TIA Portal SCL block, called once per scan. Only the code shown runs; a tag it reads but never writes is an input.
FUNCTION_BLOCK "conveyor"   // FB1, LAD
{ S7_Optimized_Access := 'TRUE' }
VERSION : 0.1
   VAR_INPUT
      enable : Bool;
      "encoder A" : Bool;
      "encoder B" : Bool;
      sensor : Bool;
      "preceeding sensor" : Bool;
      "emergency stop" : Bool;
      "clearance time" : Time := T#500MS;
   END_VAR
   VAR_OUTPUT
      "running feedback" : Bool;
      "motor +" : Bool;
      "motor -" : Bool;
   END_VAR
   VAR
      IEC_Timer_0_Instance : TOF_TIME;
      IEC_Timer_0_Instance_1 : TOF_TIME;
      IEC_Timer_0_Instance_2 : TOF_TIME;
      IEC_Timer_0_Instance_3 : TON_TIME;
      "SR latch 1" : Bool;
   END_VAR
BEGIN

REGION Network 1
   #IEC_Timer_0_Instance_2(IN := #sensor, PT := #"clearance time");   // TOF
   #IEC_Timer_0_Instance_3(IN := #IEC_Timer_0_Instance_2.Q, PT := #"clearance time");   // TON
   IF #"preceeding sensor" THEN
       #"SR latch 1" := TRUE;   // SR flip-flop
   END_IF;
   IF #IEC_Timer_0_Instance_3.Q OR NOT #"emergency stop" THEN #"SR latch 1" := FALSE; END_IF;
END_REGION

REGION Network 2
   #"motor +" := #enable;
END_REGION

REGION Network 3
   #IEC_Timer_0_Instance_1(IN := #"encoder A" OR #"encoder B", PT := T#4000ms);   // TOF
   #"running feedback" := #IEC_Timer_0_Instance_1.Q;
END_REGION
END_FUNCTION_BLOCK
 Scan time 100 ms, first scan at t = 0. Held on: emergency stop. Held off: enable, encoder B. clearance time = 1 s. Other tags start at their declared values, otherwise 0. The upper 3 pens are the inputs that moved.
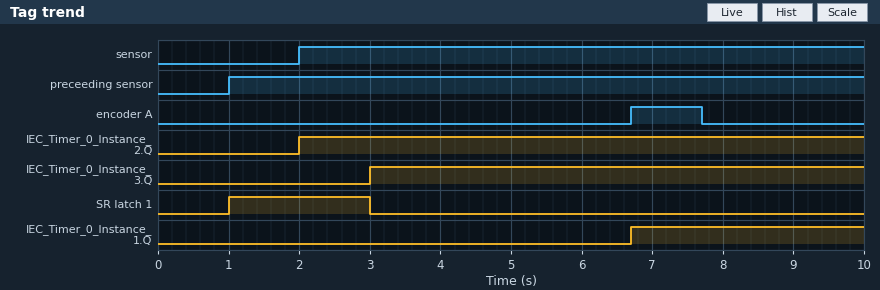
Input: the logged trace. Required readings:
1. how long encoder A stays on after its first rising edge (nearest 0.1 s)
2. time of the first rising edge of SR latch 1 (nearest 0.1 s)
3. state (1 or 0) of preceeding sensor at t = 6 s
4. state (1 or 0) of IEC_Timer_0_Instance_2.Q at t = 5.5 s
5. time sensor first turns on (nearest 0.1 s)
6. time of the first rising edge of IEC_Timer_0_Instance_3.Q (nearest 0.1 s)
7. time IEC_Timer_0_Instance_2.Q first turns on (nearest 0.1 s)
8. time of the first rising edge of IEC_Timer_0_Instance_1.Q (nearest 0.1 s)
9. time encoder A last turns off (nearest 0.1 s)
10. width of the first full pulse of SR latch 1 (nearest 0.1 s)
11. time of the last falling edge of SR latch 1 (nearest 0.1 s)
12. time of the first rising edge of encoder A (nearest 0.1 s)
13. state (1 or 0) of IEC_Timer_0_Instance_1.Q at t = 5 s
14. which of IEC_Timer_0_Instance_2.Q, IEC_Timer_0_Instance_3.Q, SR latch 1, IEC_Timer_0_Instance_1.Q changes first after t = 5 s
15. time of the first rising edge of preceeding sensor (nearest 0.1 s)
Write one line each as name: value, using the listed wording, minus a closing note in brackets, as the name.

how long encoder A stays on after its first rising edge: 1.0 s
time of the first rising edge of SR latch 1: 1.0 s
state (1 or 0) of preceeding sensor at t = 6 s: 1
state (1 or 0) of IEC_Timer_0_Instance_2.Q at t = 5.5 s: 1
time sensor first turns on: 2.0 s
time of the first rising edge of IEC_Timer_0_Instance_3.Q: 3.0 s
time IEC_Timer_0_Instance_2.Q first turns on: 2.0 s
time of the first rising edge of IEC_Timer_0_Instance_1.Q: 6.7 s
time encoder A last turns off: 7.7 s
width of the first full pulse of SR latch 1: 2.0 s
time of the last falling edge of SR latch 1: 3.0 s
time of the first rising edge of encoder A: 6.7 s
state (1 or 0) of IEC_Timer_0_Instance_1.Q at t = 5 s: 0
which of IEC_Timer_0_Instance_2.Q, IEC_Timer_0_Instance_3.Q, SR latch 1, IEC_Timer_0_Instance_1.Q changes first after t = 5 s: IEC_Timer_0_Instance_1.Q
time of the first rising edge of preceeding sensor: 1.0 s
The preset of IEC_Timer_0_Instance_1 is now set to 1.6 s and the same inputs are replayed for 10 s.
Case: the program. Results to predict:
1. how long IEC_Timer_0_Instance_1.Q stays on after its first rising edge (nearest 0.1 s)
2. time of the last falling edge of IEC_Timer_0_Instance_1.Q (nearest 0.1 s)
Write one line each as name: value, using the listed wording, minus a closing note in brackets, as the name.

how long IEC_Timer_0_Instance_1.Q stays on after its first rising edge: 2.6 s
time of the last falling edge of IEC_Timer_0_Instance_1.Q: 9.3 s
